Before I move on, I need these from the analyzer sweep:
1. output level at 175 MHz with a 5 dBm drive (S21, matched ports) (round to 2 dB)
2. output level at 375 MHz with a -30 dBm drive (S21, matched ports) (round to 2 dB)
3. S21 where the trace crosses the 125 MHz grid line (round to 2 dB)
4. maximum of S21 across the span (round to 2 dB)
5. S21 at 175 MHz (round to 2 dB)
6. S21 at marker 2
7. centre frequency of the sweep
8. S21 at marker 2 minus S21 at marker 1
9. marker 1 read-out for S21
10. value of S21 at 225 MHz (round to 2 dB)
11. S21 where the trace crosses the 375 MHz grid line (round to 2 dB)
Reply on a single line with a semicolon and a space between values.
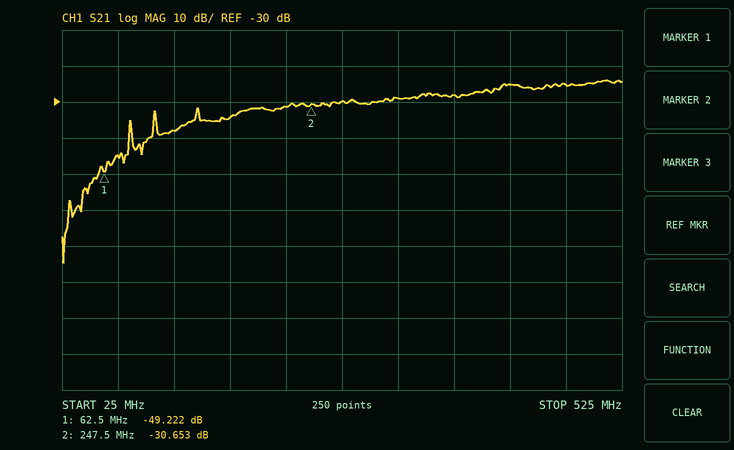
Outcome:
-30 dBm; -58 dBm; -38 dB; -24 dB; -34 dB; -30.653 dB; 275 MHz; 18.569 dB; -49.222 dB; -32 dB; -28 dB
